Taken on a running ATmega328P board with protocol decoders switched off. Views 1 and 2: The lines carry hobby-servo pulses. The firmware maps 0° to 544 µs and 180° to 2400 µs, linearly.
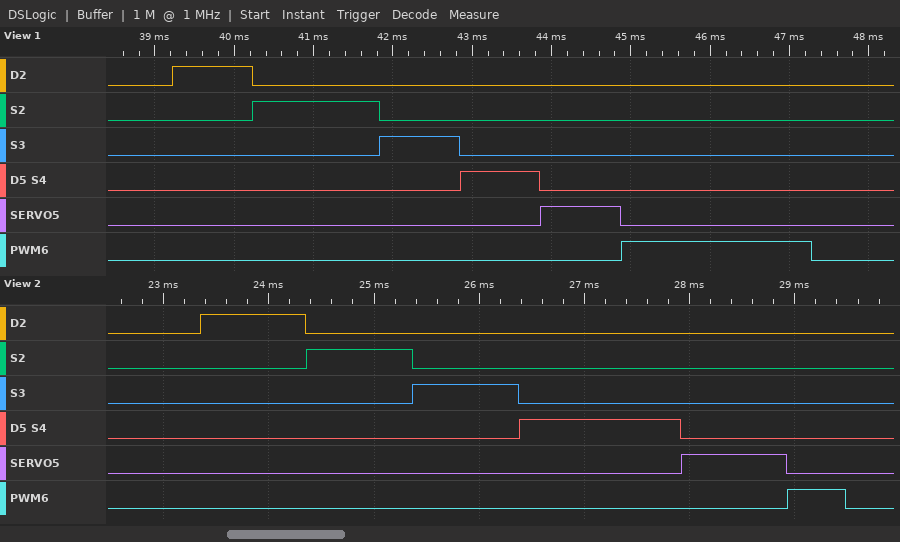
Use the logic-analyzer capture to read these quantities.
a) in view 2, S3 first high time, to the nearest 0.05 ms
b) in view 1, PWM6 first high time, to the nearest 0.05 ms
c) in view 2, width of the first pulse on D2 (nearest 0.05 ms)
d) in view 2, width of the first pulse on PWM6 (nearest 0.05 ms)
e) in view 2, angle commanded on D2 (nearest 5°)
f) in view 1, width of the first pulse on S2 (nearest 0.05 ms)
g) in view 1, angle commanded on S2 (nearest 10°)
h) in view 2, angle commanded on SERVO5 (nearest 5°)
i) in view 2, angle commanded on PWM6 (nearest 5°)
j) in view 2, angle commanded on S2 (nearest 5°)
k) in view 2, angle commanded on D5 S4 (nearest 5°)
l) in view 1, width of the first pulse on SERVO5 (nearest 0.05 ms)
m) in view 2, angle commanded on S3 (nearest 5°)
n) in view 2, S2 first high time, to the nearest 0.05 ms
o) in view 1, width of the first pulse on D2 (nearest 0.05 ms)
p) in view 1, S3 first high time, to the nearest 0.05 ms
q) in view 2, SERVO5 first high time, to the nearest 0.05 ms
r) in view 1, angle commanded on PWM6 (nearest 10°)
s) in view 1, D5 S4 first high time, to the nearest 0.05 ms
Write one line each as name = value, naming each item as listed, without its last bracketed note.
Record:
in view 2, S3 first high time, to the nearest 0.05 ms = 1.00 ms
in view 1, PWM6 first high time, to the nearest 0.05 ms = 2.40 ms
in view 2, width of the first pulse on D2 = 1.00 ms
in view 2, width of the first pulse on PWM6 = 0.55 ms
in view 2, angle commanded on D2 = 45°
in view 1, width of the first pulse on S2 = 1.60 ms
in view 1, angle commanded on S2 = 100°
in view 2, angle commanded on SERVO5 = 45°
in view 2, angle commanded on PWM6 = 0°
in view 2, angle commanded on S2 = 45°
in view 2, angle commanded on D5 S4 = 95°
in view 1, width of the first pulse on SERVO5 = 1.00 ms
in view 2, angle commanded on S3 = 45°
in view 2, S2 first high time, to the nearest 0.05 ms = 1.00 ms
in view 1, width of the first pulse on D2 = 1.00 ms
in view 1, S3 first high time, to the nearest 0.05 ms = 1.00 ms
in view 2, SERVO5 first high time, to the nearest 0.05 ms = 1.00 ms
in view 1, angle commanded on PWM6 = 180°
in view 1, D5 S4 first high time, to the nearest 0.05 ms = 1.00 ms
